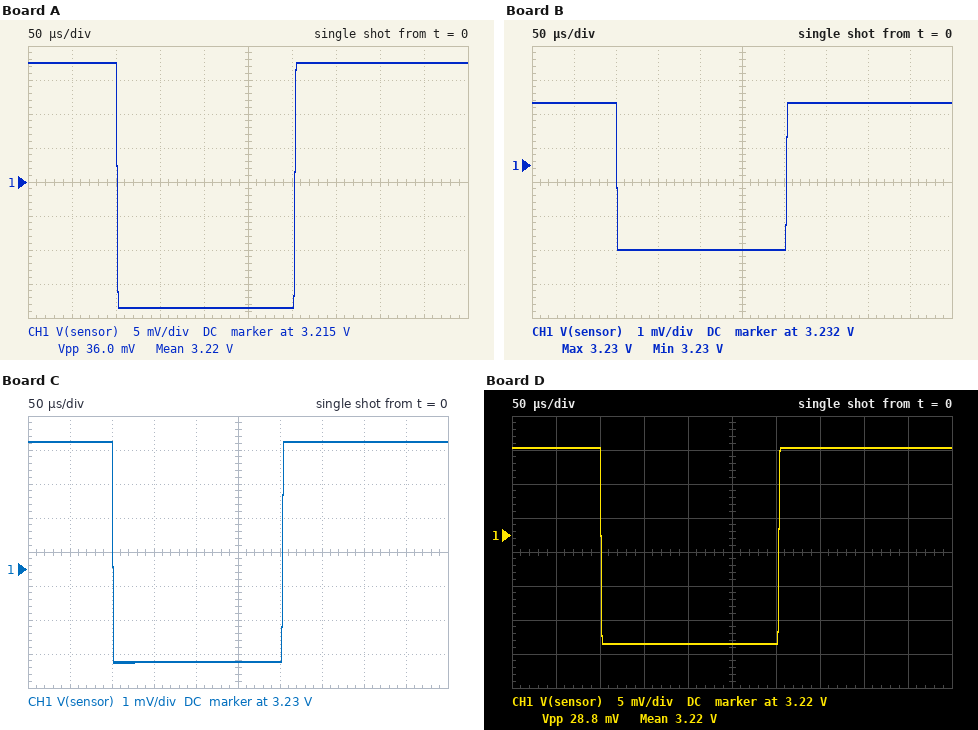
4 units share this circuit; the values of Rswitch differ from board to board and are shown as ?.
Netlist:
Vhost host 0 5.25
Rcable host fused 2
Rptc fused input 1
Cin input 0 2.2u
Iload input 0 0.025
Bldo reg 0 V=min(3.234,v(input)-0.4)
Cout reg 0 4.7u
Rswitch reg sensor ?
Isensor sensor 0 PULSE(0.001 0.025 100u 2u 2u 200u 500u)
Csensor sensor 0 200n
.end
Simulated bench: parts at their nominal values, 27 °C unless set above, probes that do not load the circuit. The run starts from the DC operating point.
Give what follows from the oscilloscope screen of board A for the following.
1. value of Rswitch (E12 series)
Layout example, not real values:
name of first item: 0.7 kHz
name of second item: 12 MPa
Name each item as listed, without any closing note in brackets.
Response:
value of Rswitch: 1.5 Ω
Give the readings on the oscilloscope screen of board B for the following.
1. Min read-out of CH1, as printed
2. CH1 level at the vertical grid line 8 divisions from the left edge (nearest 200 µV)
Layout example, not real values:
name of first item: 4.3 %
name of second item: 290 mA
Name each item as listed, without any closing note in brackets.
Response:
Min read-out of CH1, as printed: 3.23 V
CH1 level at the vertical grid line 8 divisions from the left edge: 3.2338 V
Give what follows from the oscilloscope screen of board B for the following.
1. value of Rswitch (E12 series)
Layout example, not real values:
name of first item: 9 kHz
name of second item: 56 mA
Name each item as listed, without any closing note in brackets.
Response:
value of Rswitch: 0.18 Ω
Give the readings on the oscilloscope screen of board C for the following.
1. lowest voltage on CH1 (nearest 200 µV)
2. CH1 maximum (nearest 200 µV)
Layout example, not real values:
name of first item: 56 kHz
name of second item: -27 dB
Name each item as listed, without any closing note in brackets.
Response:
lowest voltage on CH1: 3.2272 V
CH1 maximum: 3.2338 V
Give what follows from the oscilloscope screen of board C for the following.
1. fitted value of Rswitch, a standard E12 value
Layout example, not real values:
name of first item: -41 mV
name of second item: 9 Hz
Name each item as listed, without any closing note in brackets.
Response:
fitted value of Rswitch, a standard E12 value: 0.27 Ω
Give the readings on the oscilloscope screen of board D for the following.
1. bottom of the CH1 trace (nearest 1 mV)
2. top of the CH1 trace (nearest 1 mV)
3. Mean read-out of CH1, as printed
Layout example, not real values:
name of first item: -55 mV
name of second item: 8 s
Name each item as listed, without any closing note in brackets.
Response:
bottom of the CH1 trace: 3.204 V
top of the CH1 trace: 3.233 V
Mean read-out of CH1, as printed: 3.22 V
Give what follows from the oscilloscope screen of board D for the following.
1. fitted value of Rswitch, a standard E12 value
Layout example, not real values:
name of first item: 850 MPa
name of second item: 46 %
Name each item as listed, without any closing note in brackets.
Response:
fitted value of Rswitch, a standard E12 value: 1.2 Ω
